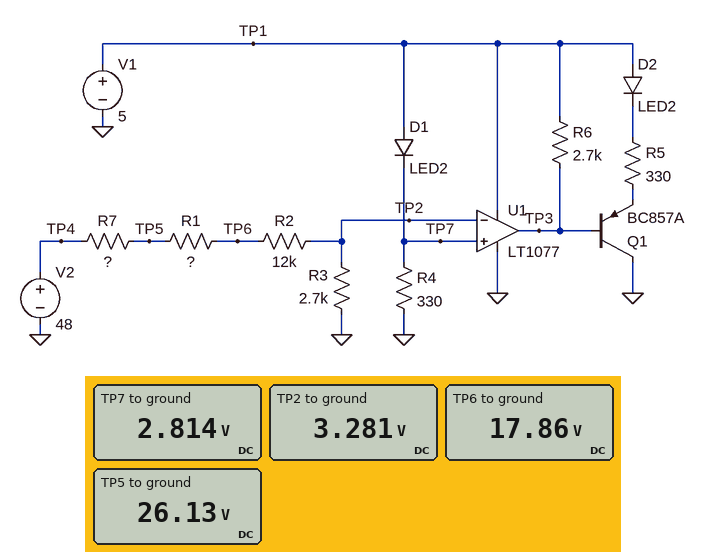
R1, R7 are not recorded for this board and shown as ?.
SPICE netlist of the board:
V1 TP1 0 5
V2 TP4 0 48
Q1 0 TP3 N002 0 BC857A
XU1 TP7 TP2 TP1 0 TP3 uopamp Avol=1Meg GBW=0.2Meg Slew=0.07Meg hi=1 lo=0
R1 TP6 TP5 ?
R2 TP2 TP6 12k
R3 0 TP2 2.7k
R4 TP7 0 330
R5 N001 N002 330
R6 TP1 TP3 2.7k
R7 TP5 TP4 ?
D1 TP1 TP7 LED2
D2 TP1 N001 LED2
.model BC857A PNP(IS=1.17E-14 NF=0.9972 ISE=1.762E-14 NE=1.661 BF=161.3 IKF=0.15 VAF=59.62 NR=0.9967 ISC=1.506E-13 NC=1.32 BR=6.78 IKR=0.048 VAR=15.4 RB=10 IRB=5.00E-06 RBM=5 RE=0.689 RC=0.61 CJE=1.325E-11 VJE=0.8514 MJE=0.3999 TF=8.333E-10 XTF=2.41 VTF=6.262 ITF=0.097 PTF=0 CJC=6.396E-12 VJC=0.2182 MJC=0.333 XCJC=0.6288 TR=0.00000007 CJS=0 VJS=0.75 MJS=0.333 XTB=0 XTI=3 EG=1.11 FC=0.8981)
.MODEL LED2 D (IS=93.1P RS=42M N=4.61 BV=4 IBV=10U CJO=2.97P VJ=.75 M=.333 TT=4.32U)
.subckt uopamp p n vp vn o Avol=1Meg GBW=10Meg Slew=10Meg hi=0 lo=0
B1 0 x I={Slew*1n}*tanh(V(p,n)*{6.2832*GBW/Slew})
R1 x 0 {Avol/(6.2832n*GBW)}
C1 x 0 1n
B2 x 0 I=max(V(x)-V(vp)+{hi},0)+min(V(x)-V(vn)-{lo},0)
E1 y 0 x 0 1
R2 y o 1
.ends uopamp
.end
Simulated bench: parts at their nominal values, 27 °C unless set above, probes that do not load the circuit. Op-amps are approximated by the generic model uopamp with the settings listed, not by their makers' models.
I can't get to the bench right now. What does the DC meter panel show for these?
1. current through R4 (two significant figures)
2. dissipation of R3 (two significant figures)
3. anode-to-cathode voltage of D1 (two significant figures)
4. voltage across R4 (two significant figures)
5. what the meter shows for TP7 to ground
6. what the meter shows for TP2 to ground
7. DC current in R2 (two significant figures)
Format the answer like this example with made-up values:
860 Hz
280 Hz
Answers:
8.5 mA
4.0 mW
2.2 V
2.8 V
2.814 V
3.281 V
1.2 mA
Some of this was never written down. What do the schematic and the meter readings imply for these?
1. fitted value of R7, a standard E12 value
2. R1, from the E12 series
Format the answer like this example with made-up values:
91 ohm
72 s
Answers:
18 kΩ
6.8 kΩ
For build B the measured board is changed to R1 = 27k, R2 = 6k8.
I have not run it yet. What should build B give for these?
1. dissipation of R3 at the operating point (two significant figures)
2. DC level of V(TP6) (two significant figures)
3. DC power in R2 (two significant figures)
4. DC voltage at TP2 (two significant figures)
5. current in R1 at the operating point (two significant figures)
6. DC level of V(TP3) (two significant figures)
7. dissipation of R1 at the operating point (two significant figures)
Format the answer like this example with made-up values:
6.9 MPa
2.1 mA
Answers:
2.1 mW
8.4 V
5.3 mW
2.4 V
880 µA
4.0 V
21 mW
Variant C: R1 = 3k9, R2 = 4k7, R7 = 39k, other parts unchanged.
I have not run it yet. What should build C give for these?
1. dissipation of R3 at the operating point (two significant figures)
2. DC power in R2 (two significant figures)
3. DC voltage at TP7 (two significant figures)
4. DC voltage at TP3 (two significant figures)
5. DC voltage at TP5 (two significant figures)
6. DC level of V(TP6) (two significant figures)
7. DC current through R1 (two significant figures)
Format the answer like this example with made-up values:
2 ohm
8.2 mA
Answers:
2.5 mW
4.3 mW
2.8 V
4.0 V
11 V
7.1 V
950 µA
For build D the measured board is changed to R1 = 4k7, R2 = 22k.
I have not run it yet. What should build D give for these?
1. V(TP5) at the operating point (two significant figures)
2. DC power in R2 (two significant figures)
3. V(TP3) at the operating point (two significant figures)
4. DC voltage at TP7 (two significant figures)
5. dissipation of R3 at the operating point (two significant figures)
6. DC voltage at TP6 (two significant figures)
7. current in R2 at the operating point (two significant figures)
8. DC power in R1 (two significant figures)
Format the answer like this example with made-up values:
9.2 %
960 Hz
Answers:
30 V
23 mW
4.0 V
2.8 V
2.8 mW
25 V
1.0 mA
4.8 mW
